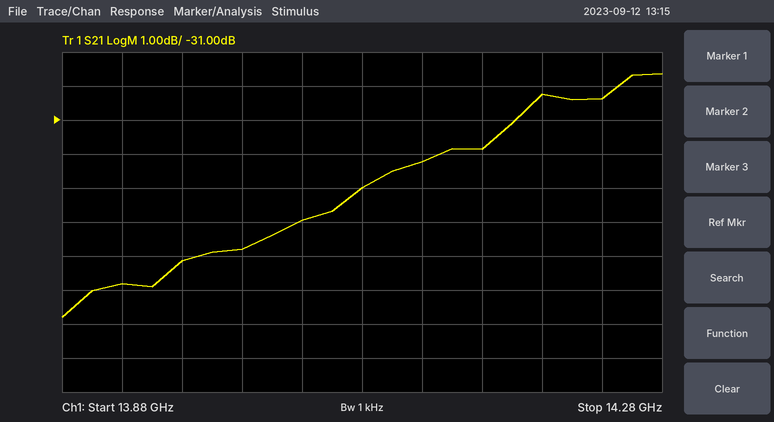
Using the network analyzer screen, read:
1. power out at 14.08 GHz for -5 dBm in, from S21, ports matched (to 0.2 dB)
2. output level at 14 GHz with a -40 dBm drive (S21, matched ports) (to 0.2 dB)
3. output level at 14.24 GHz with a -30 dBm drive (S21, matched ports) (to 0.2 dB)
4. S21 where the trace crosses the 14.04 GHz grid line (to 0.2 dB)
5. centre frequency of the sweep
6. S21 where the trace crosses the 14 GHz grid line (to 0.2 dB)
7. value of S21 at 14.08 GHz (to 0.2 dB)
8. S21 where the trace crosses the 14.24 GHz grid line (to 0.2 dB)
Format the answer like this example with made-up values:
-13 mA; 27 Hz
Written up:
-38.0 dBm; -74.8 dBm; -60.4 dBm; -34.0 dB; 14.08 GHz; -34.8 dB; -33.0 dB; -30.4 dB
